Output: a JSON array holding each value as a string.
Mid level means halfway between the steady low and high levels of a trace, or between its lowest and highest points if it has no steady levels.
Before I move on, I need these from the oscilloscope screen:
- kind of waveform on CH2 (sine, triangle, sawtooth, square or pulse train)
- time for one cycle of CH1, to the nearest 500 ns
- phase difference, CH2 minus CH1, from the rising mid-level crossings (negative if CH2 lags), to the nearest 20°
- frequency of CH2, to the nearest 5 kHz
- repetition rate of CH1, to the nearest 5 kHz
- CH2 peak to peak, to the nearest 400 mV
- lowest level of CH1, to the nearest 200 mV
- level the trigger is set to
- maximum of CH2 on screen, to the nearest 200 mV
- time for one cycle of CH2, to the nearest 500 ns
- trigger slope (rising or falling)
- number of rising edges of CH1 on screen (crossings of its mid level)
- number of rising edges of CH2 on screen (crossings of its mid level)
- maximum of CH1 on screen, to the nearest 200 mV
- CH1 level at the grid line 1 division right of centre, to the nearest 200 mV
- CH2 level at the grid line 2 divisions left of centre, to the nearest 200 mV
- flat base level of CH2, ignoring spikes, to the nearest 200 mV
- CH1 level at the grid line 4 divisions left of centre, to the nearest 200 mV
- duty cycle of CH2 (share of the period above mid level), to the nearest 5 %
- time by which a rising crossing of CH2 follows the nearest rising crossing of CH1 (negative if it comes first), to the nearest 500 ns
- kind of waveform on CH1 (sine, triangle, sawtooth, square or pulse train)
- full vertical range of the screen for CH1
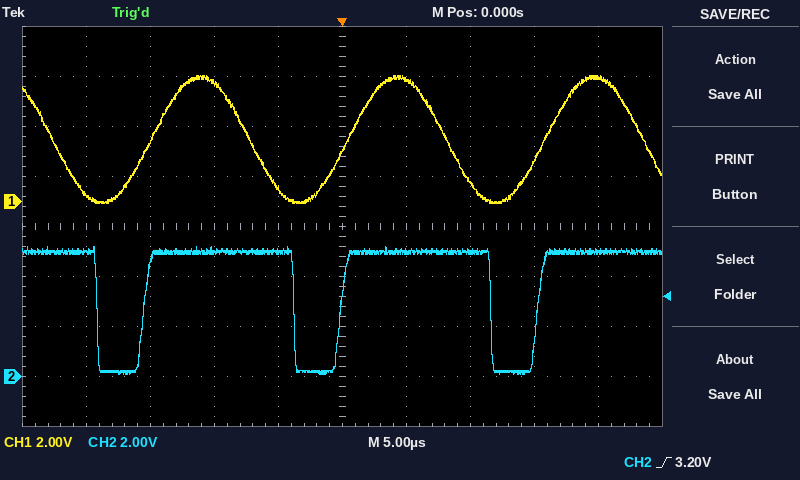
["pulse train", "15.5 µs", "+20°", "65 kHz", "65 kHz", "5.2 V", "0.0 V", "3.20 V", "5.2 V", "15.5 µs", "rising", "3", "3", "5.0 V", "4.8 V", "5.0 V", "200 mV", "200 mV", "75 %", "-500 ns", "sine", "16 V"]
